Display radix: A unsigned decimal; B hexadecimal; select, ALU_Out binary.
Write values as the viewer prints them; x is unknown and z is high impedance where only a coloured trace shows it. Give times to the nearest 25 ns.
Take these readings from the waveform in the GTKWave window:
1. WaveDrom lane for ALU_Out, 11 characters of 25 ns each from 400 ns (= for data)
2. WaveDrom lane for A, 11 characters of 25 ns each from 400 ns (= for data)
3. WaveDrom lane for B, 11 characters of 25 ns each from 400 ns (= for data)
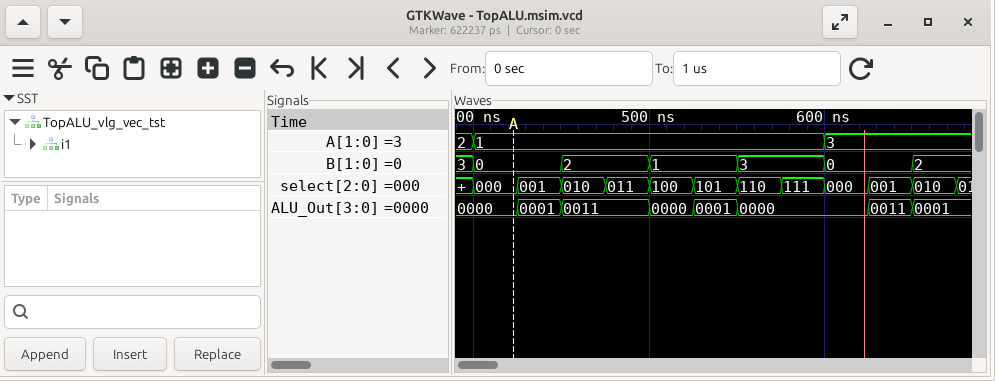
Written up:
{name: 'ALU_Out', wave: '===.===..==', data: '0000 0001 0011 0000 0001 0000 0011 0001'}
{name: 'A', wave: '=.......=..', data: '1 3'}
{name: 'B', wave: '=.=.=.=.=.=', data: '0 2 1 3 0 2'}
